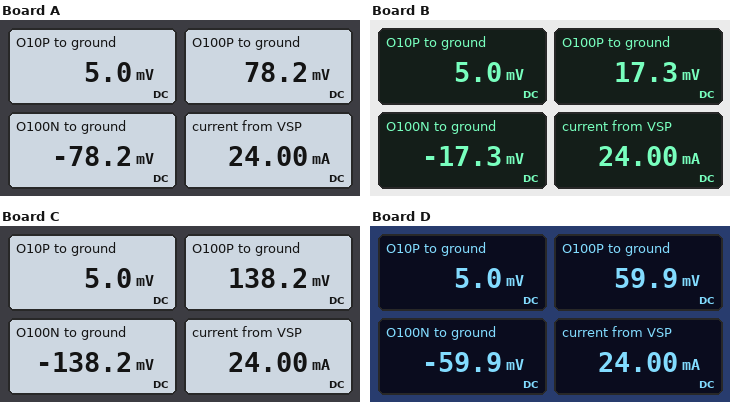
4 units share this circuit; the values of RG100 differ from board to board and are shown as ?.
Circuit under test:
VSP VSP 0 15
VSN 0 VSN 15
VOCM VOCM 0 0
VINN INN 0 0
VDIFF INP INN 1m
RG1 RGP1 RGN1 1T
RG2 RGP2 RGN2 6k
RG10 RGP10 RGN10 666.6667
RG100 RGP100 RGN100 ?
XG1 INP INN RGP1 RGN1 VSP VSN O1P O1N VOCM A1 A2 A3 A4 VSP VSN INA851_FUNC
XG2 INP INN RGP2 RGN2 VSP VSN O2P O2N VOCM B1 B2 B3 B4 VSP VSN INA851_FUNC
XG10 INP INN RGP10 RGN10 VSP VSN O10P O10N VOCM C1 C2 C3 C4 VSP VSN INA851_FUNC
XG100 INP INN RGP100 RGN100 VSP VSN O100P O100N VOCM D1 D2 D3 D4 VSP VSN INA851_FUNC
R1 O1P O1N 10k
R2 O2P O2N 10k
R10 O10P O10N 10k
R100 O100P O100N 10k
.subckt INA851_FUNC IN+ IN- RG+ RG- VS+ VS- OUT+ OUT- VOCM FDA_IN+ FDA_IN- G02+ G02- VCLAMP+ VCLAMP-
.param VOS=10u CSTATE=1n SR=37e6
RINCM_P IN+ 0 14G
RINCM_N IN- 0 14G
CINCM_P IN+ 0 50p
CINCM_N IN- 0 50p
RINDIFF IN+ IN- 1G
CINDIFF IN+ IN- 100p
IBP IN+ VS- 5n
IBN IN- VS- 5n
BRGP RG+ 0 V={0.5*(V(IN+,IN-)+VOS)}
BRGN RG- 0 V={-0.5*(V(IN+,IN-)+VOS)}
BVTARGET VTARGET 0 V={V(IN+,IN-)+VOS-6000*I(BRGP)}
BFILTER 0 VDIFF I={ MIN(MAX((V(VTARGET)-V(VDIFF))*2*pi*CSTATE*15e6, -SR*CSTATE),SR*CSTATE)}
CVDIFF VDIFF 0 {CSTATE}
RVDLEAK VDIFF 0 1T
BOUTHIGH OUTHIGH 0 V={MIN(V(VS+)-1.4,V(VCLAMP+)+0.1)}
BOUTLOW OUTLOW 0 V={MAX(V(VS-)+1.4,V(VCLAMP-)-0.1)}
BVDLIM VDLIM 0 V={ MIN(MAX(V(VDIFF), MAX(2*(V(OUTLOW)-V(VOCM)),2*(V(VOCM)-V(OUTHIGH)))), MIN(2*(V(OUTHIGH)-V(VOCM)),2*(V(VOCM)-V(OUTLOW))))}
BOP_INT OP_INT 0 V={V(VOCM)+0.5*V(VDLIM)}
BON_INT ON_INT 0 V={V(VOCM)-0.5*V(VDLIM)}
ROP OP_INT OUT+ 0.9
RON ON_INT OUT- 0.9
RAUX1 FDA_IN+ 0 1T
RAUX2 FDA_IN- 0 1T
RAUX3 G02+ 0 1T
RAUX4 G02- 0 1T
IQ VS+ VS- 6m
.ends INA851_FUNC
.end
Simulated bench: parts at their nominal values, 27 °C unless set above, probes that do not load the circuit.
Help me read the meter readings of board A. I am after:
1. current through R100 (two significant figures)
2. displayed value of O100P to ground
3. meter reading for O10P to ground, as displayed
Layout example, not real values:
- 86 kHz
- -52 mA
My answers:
- 16 µA
- 78.2 mV
- 5.0 mV
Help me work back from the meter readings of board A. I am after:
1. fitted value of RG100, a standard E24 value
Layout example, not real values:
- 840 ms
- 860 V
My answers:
- 39 Ω
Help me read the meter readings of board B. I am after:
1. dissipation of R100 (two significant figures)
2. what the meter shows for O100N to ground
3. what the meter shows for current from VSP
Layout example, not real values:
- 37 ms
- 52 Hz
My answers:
- 120 nW
- -17.3 mV
- 24.00 mA
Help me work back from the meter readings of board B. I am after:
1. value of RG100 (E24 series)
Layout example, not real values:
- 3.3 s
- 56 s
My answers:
- 180 Ω
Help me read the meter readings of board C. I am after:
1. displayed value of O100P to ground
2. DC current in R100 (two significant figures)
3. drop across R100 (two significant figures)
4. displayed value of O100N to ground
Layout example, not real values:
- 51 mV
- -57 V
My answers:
- 138.2 mV
- 28 µA
- 280 mV
- -138.2 mV
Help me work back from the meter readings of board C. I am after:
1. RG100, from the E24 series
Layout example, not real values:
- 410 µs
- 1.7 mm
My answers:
- 22 Ω
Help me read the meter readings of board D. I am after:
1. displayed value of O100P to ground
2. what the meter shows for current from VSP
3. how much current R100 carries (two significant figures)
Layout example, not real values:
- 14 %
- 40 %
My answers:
- 59.9 mV
- 24.00 mA
- 12 µA
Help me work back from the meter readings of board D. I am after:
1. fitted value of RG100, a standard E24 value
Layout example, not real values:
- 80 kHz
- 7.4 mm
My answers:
- 51 Ω
